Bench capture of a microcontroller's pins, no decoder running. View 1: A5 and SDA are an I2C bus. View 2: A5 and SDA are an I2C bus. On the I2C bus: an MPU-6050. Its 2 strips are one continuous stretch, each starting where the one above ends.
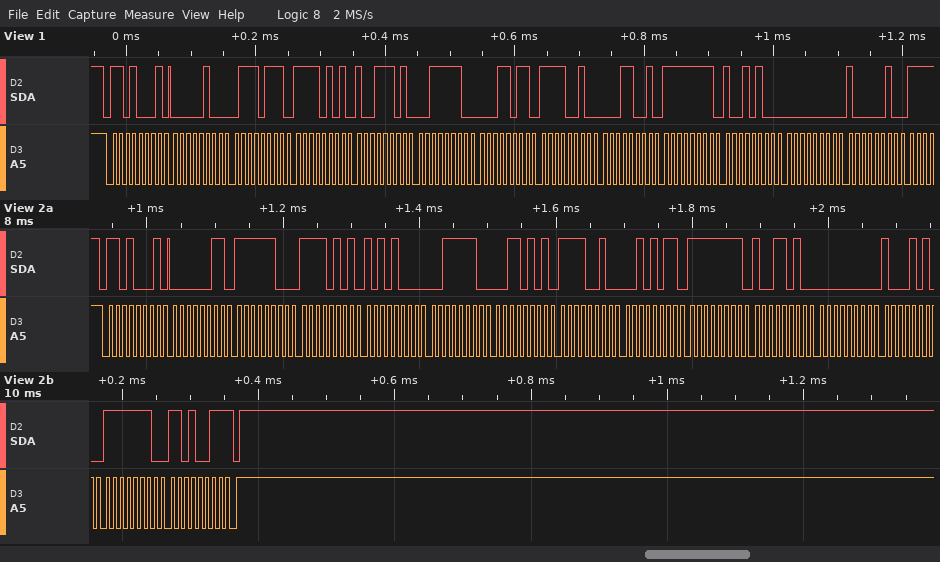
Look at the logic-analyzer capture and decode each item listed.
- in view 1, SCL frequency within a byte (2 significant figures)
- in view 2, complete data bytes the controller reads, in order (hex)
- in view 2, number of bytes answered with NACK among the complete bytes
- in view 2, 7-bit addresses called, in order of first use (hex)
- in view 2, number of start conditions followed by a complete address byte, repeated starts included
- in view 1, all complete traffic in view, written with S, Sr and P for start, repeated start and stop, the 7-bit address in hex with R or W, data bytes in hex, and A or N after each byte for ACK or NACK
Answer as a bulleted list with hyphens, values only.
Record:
- 100 kHz
- 03 FC F5 A8 3E 35 F2 2B FF 9A 00 8A FE D3
- 1
- 0x68
- 1
- S 68R A 04 A 77 A F5 A 9D A 3E A 1B A F2 A 19 A FF A 94 A 00 A 82 A
